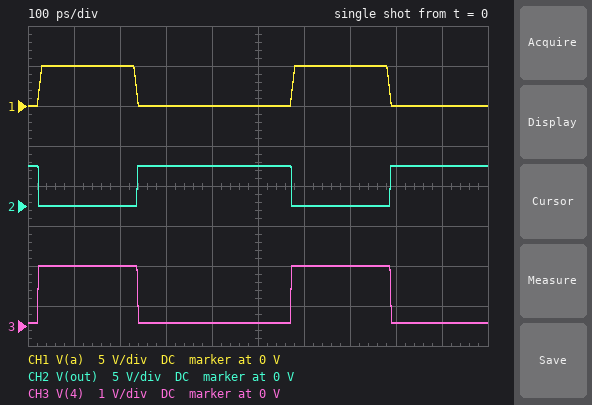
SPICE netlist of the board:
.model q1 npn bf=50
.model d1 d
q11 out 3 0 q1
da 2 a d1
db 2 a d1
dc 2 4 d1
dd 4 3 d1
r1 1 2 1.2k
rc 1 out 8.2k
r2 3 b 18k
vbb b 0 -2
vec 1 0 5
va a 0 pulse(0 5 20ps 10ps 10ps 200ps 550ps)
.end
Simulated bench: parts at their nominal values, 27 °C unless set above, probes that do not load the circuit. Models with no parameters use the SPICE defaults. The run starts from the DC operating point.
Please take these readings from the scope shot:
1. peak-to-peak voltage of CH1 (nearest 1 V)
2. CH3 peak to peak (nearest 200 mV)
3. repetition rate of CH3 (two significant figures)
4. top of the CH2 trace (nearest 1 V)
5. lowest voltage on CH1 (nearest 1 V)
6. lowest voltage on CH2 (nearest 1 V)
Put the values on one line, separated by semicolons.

5 V; 1.4 V; 1.8 GHz; 5 V; 0 V; 0 V
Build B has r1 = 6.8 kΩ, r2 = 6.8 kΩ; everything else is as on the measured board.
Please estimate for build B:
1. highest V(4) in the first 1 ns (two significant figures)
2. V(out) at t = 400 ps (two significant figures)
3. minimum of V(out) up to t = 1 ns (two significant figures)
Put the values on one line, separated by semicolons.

1.4 V; 5.0 V; 92 mV
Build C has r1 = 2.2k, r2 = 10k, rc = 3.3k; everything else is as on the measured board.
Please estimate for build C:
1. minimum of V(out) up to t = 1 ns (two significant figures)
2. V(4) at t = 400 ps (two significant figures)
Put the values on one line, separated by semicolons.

33 mV; 48 mV
